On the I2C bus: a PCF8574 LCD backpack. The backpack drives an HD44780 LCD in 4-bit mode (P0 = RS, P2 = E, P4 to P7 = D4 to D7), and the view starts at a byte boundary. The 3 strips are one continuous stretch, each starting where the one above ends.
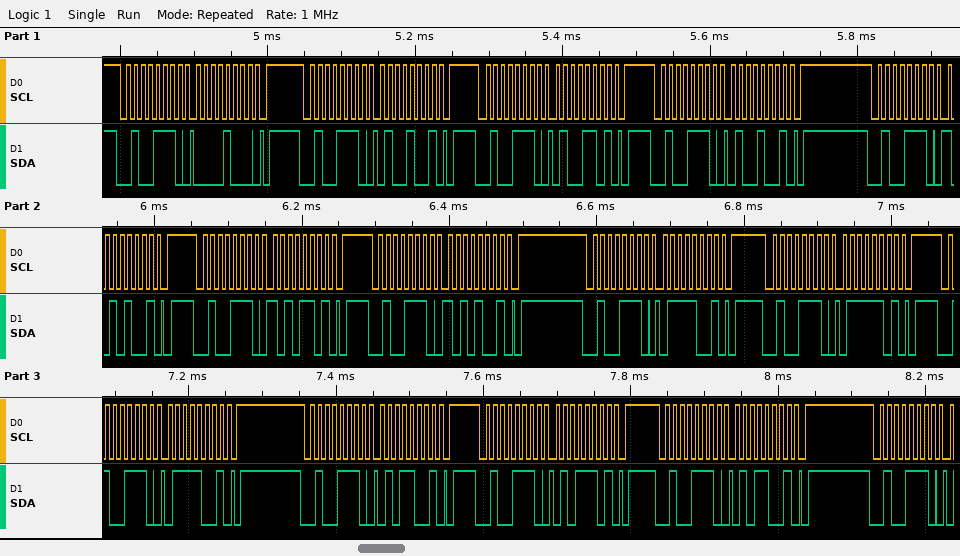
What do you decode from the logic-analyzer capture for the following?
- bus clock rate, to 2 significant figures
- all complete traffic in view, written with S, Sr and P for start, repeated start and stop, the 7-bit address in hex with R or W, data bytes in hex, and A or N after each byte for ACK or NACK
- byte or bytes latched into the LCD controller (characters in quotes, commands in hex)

100 kHz
S 27W A 08 A P S 27W A 49 A P S 27W A 4D A P S 27W A 49 A P S 27W A A9 A P S 27W A AD A P S 27W A A9 A P S 27W A 79 A P S 27W A 7D A P S 27W A 79 A P S 27W A 59 A P S 27W A 5D A P S 27W A 59 A P S 27W A
'J' 'u'
